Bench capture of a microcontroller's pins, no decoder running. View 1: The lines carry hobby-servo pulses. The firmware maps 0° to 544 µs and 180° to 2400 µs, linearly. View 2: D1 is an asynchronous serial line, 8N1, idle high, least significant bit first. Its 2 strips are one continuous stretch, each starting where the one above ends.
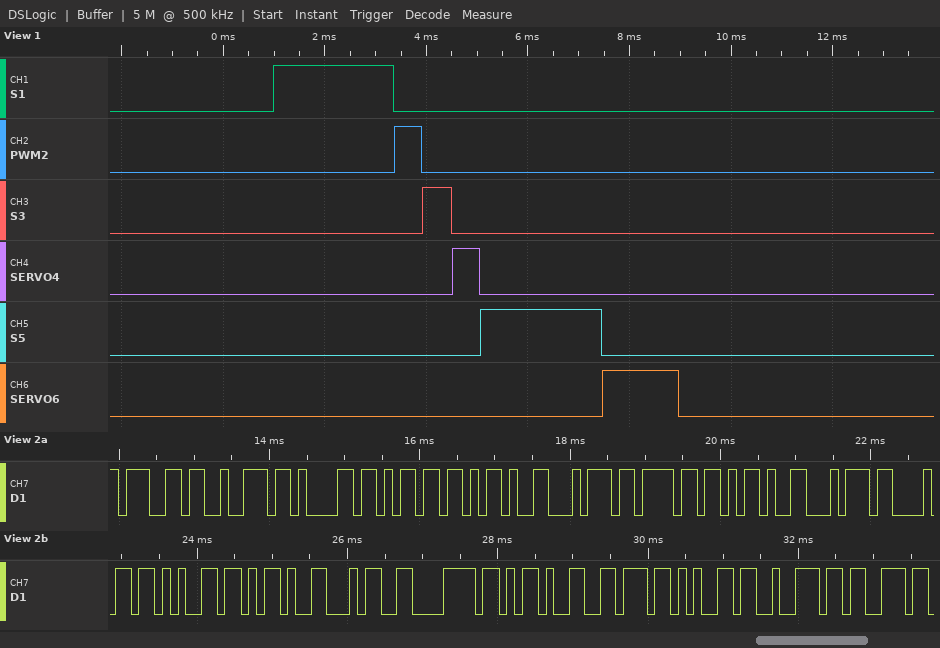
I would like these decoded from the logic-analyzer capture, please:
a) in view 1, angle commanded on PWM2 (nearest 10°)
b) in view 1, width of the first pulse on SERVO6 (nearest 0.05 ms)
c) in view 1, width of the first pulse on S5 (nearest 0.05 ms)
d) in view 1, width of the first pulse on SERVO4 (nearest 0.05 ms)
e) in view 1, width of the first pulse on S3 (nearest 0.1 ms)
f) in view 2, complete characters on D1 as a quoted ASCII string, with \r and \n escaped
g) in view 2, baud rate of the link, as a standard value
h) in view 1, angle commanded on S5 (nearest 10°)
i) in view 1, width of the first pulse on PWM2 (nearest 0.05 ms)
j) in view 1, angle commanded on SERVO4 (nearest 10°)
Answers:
0°
1.50 ms
2.40 ms
0.55 ms
0.6 ms
"gram-to-the-4x-vers"
9600 baud
180°
0.55 ms
0°
